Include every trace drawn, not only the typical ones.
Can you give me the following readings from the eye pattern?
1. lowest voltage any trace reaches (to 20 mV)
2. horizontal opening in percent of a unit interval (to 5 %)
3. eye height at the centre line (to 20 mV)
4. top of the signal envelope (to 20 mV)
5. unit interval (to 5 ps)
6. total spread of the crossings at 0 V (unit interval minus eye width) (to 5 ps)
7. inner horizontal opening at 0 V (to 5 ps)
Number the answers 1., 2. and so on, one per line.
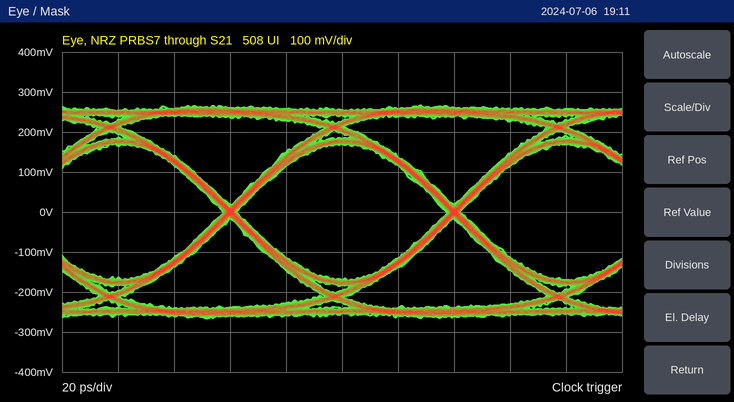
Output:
1. -260 mV
2. 95 %
3. 340 mV
4. 260 mV
5. 80 ps
6. 5 ps
7. 75 ps
